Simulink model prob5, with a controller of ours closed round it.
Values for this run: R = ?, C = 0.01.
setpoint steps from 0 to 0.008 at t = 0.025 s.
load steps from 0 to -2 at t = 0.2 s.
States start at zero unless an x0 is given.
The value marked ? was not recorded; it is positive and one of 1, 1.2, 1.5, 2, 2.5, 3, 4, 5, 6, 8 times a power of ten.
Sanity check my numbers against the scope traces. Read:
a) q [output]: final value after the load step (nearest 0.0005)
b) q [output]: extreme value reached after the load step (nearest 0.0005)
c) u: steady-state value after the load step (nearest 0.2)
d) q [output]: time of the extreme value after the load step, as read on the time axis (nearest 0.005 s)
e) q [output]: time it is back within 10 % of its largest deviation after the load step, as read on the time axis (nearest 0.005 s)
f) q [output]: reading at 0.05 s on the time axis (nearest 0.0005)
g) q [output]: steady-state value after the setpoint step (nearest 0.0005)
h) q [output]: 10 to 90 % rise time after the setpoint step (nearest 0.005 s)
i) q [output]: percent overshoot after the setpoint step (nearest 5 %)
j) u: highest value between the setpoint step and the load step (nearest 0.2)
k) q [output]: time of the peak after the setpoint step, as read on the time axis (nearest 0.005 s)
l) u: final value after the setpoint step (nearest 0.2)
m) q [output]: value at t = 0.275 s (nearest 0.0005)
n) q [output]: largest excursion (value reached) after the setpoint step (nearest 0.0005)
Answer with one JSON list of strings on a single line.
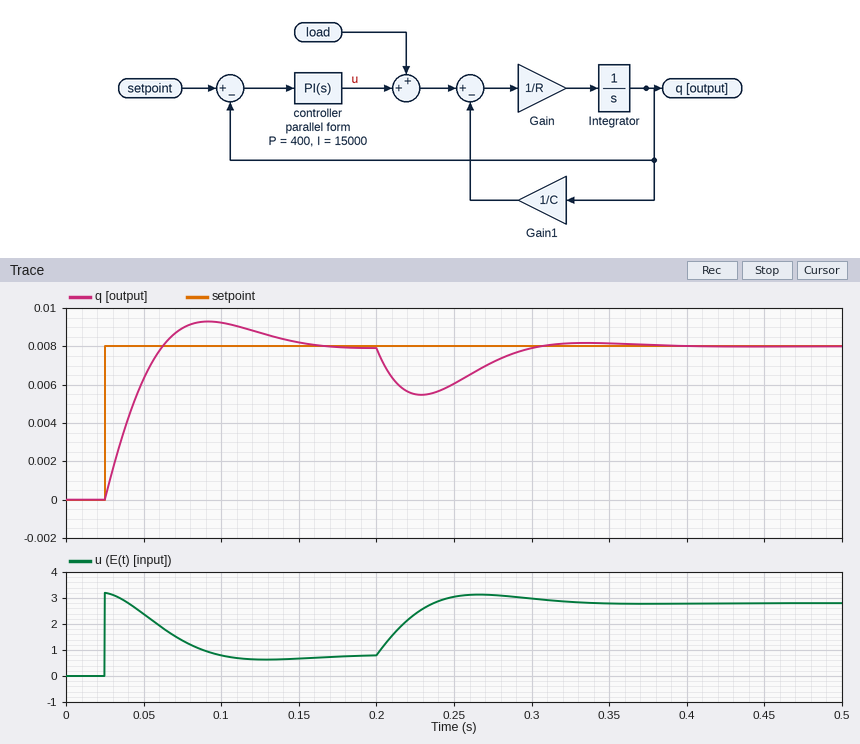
["0.0080", "0.0055", "2.8", "0.230 s", "0.295 s", "0.0065", "0.0080", "0.030 s", "15 %", "3.2", "0.090 s", "0.8", "0.0070", "0.0095"]
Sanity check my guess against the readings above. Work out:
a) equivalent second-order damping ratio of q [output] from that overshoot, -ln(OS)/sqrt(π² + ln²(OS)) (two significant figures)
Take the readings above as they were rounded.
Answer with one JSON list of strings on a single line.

["0.52"]
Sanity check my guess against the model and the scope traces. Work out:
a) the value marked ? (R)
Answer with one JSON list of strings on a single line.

["10"]
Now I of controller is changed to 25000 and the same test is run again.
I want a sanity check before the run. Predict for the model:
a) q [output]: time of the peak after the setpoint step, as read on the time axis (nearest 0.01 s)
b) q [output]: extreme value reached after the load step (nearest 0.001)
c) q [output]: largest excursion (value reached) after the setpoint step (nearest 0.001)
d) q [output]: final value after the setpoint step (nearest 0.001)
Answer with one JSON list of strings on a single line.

["0.08 s", "0.006", "0.010", "0.008"]
